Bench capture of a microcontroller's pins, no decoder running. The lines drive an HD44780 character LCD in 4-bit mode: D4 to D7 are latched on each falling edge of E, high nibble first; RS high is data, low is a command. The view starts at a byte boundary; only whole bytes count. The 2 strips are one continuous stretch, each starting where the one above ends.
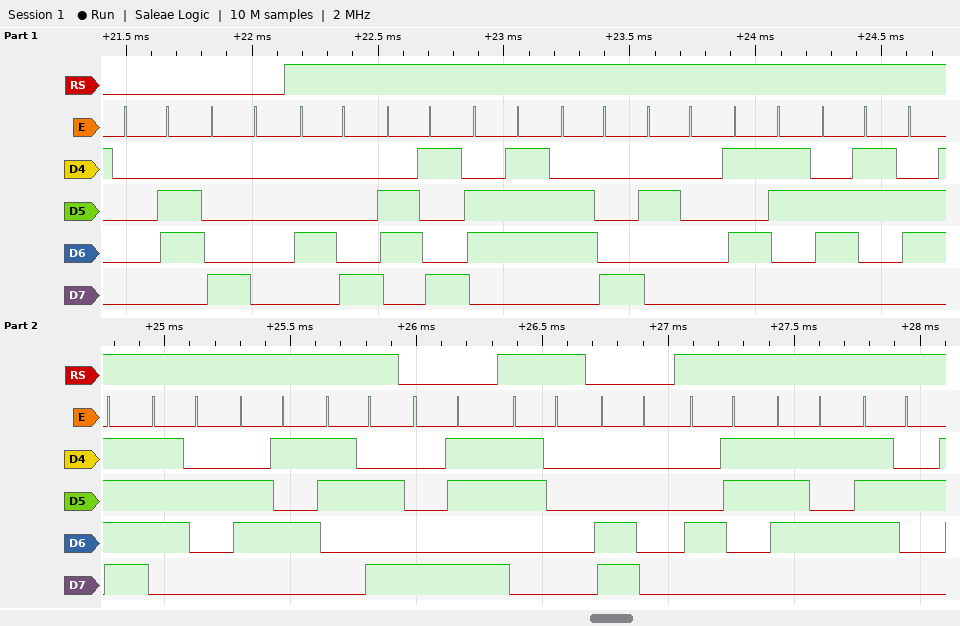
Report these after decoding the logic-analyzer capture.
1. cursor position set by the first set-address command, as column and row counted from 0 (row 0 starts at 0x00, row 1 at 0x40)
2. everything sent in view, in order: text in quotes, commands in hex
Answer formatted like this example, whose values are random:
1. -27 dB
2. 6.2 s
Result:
1. column 0, row 0
2. 0x06 0x80 "High Score:" 0x8B "0" 0xC0 "Cur"
